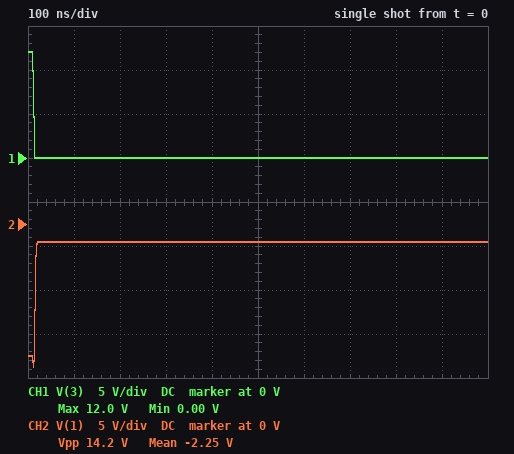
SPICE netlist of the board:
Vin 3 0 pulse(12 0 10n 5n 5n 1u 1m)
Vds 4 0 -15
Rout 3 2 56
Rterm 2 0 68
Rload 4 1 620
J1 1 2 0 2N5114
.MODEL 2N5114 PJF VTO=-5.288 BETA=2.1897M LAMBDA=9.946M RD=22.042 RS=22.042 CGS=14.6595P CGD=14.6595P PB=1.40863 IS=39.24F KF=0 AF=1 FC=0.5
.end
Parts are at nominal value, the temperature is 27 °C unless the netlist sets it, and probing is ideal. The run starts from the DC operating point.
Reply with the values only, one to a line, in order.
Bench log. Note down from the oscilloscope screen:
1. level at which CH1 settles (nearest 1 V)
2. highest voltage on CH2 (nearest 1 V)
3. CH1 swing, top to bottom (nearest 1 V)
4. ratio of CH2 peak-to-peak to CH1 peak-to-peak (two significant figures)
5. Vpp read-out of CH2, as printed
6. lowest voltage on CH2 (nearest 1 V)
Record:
0 V
-2 V
12 V
1.2
14.2 V
-16 V
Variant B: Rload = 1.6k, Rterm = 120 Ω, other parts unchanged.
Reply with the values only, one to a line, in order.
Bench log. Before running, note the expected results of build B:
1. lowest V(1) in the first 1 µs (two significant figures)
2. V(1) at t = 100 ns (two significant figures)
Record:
-18 V
-800 mV
